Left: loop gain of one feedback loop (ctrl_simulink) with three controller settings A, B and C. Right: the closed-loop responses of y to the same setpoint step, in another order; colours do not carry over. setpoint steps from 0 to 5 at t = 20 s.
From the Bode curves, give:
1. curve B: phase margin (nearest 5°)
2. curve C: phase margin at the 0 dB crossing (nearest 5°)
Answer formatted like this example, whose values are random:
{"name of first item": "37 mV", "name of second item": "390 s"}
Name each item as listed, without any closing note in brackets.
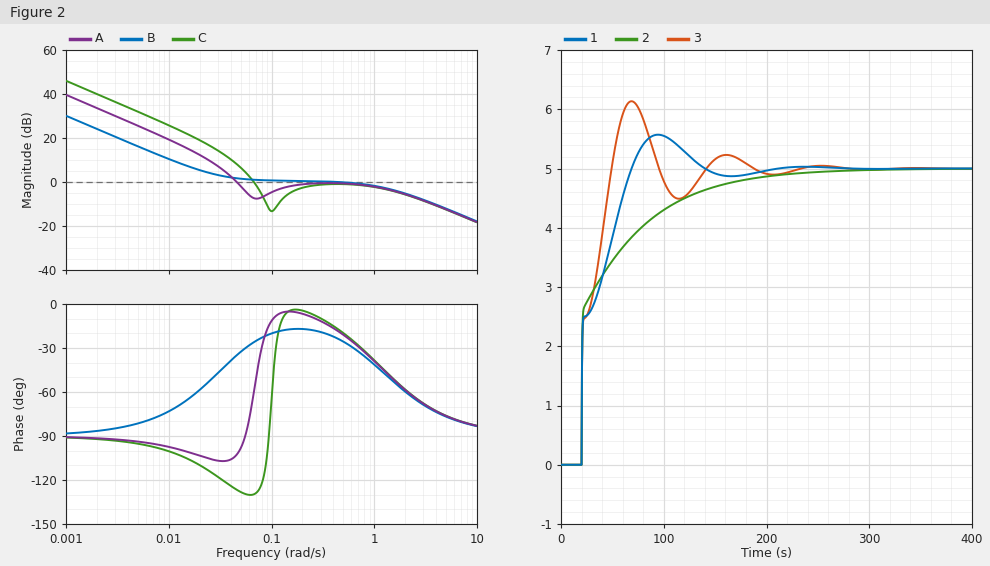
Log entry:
{"curve B: phase margin": "155°", "curve C: phase margin at the 0 dB crossing": "50°"}
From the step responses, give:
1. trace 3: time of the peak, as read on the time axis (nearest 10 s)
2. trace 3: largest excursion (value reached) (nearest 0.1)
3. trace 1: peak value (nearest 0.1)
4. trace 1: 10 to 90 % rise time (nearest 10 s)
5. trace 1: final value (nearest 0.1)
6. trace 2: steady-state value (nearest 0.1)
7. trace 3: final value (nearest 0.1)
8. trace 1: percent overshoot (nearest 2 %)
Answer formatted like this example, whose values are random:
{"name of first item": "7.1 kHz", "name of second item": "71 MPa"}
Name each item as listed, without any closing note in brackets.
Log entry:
{"trace 3: time of the peak, as read on the time axis": "70 s", "trace 3: largest excursion (value reached)": "6.1", "trace 1: peak value": "5.6", "trace 1: 10 to 90 % rise time": "40 s", "trace 1: final value": "5.0", "trace 2: steady-state value": "5.0", "trace 3: final value": "5.0", "trace 1: percent overshoot": "12 %"}
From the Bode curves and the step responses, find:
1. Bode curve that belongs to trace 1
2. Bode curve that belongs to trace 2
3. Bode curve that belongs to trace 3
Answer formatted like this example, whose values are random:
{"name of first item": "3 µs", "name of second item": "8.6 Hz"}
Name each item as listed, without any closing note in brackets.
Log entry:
{"Bode curve that belongs to trace 1": "A", "Bode curve that belongs to trace 2": "B", "Bode curve that belongs to trace 3": "C"}
